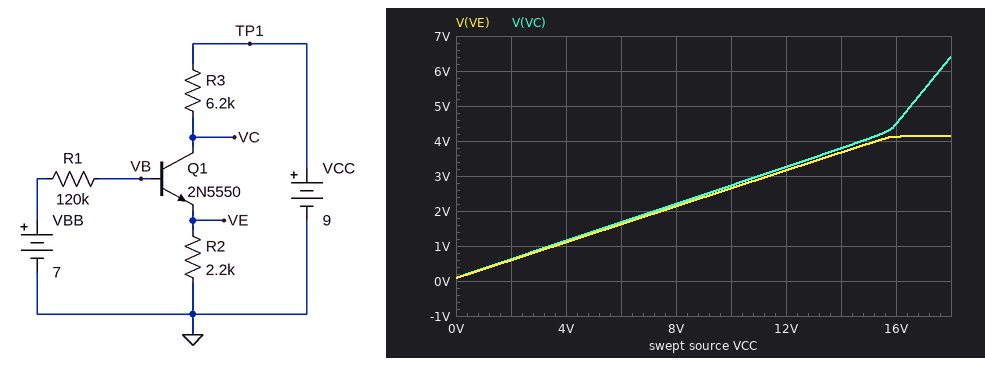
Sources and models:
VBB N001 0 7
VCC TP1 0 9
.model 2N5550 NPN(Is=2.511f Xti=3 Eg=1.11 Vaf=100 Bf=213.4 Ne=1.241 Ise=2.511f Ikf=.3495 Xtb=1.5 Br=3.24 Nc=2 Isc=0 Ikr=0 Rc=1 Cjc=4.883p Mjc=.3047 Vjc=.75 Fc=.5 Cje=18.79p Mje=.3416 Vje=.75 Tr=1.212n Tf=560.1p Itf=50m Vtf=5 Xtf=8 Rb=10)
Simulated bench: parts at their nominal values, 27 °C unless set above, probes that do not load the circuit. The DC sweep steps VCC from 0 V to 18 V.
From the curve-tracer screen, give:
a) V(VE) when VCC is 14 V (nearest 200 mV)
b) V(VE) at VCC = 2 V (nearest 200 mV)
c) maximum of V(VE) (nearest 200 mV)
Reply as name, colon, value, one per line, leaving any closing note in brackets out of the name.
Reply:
V(VE) when VCC is 14 V: 3.6 V
V(VE) at VCC = 2 V: 600 mV
maximum of V(VE): 4.2 V
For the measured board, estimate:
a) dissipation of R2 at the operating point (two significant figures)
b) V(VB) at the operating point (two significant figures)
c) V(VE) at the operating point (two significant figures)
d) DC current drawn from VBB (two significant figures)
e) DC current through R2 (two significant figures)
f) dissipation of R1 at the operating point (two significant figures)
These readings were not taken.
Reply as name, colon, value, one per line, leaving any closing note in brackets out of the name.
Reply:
dissipation of R2 at the operating point: 2.6 mW
V(VB) at the operating point: 3.1 V
V(VE) at the operating point: 2.4 V
DC current drawn from VBB: 33 µA
DC current through R2: 1.1 mA
dissipation of R1 at the operating point: 130 µW
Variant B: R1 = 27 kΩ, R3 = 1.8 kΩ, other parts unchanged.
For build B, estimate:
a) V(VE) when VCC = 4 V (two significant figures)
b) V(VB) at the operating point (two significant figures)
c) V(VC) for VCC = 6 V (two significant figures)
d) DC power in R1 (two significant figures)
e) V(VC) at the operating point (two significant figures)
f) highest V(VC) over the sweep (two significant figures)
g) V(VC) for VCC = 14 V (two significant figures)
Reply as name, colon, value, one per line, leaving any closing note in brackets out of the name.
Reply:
V(VE) when VCC = 4 V: 2.3 V
V(VB) at the operating point: 5.7 V
V(VC) for VCC = 6 V: 3.4 V
DC power in R1: 66 µW
V(VC) at the operating point: 5.0 V
highest V(VC) over the sweep: 13 V
V(VC) for VCC = 14 V: 9.4 V
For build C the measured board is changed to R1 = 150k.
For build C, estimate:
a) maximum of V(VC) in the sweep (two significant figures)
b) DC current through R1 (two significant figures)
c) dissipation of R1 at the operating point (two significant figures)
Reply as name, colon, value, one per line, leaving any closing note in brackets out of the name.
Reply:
maximum of V(VC) in the sweep: 7.3 V
DC current through R1: 26 µA
dissipation of R1 at the operating point: 100 µW
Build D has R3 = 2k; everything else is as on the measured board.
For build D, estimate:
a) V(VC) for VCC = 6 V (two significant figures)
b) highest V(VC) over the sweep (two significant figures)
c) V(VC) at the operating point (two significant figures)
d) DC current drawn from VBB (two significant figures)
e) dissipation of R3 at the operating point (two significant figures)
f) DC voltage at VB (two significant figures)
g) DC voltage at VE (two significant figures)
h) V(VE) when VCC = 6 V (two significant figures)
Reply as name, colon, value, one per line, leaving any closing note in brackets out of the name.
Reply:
V(VC) for VCC = 6 V: 3.2 V
highest V(VC) over the sweep: 14 V
V(VC) at the operating point: 5.3 V
DC current drawn from VBB: 18 µA
dissipation of R3 at the operating point: 6.9 mW
DC voltage at VB: 4.8 V
DC voltage at VE: 4.1 V
V(VE) when VCC = 6 V: 3.1 V
